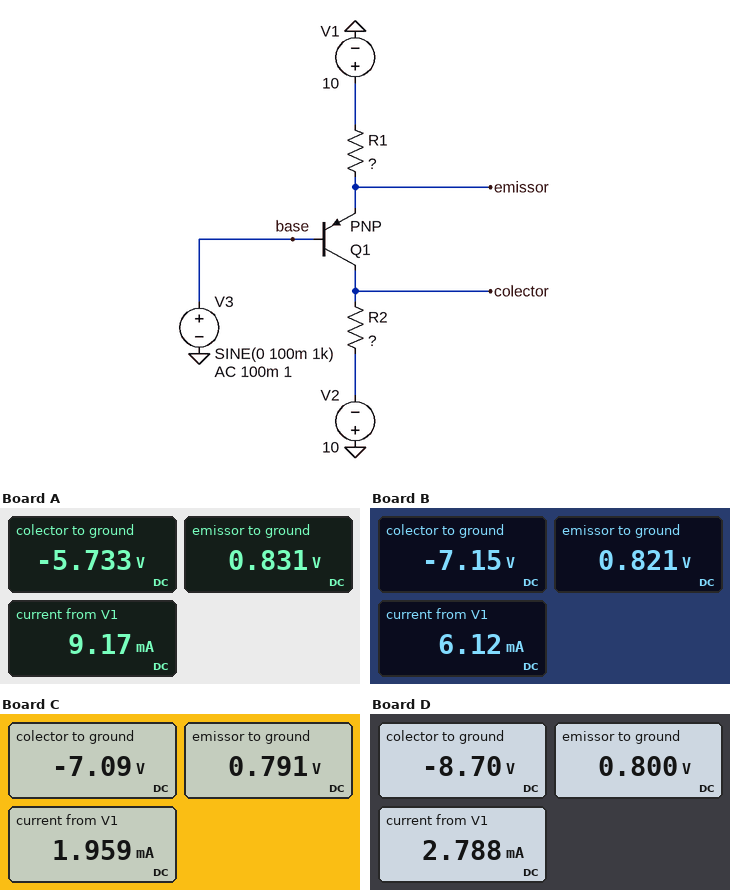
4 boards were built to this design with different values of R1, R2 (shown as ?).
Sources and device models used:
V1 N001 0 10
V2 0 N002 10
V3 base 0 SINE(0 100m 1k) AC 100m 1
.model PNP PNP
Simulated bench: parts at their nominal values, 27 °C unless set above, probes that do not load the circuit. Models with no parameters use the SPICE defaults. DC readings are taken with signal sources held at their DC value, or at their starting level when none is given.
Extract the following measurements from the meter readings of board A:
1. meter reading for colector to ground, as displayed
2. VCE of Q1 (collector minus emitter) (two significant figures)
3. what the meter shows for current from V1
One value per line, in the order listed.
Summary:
-5.733 V
-6.6 V
9.17 mA
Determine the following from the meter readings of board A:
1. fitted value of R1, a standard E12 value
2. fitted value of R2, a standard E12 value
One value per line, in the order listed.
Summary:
1 kΩ
470 Ω
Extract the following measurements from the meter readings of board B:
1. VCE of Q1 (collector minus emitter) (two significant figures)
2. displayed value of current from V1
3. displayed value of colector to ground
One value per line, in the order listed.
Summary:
-8.0 V
6.12 mA
-7.15 V
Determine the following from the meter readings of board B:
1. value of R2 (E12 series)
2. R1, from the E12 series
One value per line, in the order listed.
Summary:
470 Ω
1.5 kΩ
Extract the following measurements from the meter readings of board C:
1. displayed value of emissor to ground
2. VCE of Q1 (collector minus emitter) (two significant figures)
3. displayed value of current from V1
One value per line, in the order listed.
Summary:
0.791 V
-7.9 V
1.959 mA
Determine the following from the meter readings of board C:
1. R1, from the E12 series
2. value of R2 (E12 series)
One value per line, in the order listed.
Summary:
4.7 kΩ
1.5 kΩ
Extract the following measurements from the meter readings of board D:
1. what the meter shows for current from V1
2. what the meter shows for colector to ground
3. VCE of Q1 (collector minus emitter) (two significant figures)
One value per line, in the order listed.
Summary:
2.788 mA
-8.70 V
-9.5 V
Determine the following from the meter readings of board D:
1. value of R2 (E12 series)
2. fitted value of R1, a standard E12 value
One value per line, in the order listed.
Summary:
470 Ω
3.3 kΩ
